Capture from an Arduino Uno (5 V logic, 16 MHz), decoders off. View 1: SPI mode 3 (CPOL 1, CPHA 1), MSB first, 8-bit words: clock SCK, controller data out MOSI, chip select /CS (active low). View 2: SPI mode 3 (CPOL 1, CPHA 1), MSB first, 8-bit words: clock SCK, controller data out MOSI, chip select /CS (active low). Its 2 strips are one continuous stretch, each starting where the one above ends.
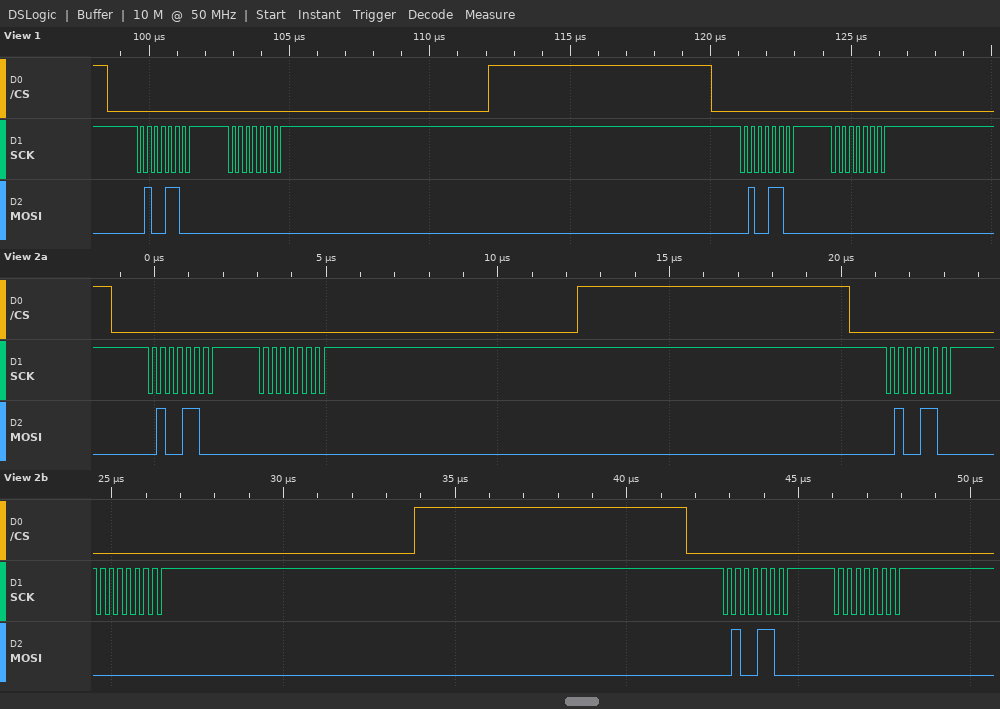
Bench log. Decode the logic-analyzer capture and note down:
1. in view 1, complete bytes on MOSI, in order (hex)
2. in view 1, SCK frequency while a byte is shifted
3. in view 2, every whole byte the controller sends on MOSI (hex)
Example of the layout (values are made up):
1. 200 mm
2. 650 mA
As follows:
1. 4C 00 4C 00
2. 4 MHz
3. 4C 00 4C 00 4C 00
